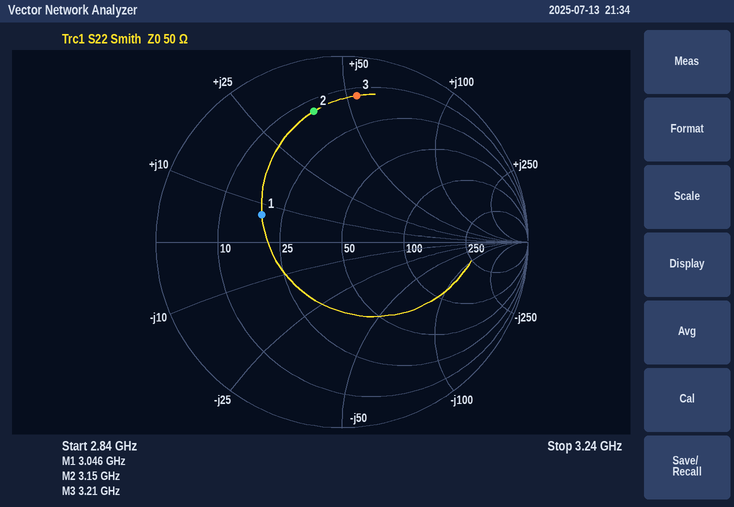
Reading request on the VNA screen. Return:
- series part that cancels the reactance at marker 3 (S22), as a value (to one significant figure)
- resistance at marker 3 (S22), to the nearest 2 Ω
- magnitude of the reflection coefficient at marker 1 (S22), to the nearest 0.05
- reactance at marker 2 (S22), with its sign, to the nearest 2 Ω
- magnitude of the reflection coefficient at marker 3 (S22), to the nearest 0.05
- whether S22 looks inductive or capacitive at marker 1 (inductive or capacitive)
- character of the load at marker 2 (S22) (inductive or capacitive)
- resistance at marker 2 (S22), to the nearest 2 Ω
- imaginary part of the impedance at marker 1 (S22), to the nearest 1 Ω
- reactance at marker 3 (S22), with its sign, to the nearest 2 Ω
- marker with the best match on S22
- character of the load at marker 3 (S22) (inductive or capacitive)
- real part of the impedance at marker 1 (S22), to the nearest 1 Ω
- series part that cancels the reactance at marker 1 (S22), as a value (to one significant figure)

900 fF
12 Ω
0.45
+38 Ω
0.80
inductive
inductive
14 Ω
+7 Ω
+54 Ω
marker 1
inductive
19 Ω
7 pF
